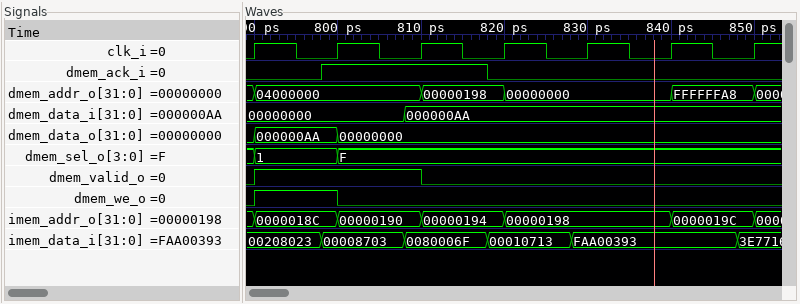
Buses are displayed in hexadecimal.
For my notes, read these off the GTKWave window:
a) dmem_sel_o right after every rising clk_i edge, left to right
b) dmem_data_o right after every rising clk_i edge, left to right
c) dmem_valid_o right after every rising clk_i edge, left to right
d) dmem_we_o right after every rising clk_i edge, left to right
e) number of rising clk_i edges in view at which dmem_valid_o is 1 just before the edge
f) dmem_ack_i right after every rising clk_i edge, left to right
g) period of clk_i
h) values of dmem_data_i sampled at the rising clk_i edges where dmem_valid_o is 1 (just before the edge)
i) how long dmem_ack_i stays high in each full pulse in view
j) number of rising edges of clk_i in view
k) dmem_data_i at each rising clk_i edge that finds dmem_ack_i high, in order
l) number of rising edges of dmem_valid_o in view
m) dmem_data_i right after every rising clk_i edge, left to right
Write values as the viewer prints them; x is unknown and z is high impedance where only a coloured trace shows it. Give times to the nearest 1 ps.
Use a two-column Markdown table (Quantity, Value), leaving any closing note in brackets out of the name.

| Quantity | Value |
|---|---|
| dmem_sel_o right after every rising clk_i edge, left to right | 1, F, F, F, F, F, F |
| dmem_data_o right after every rising clk_i edge, left to right | 000000AA, 00000000, 00000000, 00000000, 00000000, 00000000, 00000000 |
| dmem_valid_o right after every rising clk_i edge, left to right | 1 1 0 0 0 0 0 |
| dmem_we_o right after every rising clk_i edge, left to right | 1 0 0 0 0 0 0 |
| number of rising clk_i edges in view at which dmem_valid_o is 1 just before the edge | 2 |
| dmem_ack_i right after every rising clk_i edge, left to right | 0 1 1 0 0 0 0 |
| period of clk_i | 10 ps |
| values of dmem_data_i sampled at the rising clk_i edges where dmem_valid_o is 1 | 00000000, 000000AA |
| how long dmem_ack_i stays high in each full pulse in view | 20 ps |
| number of rising edges of clk_i in view | 7 |
| dmem_data_i at each rising clk_i edge that finds dmem_ack_i high, in order | 00000000, 000000AA |
| number of rising edges of dmem_valid_o in view | 1 |
| dmem_data_i right after every rising clk_i edge, left to right | 00000000, 00000000, 000000AA, 000000AA, 000000AA, 000000AA, 000000AA |
